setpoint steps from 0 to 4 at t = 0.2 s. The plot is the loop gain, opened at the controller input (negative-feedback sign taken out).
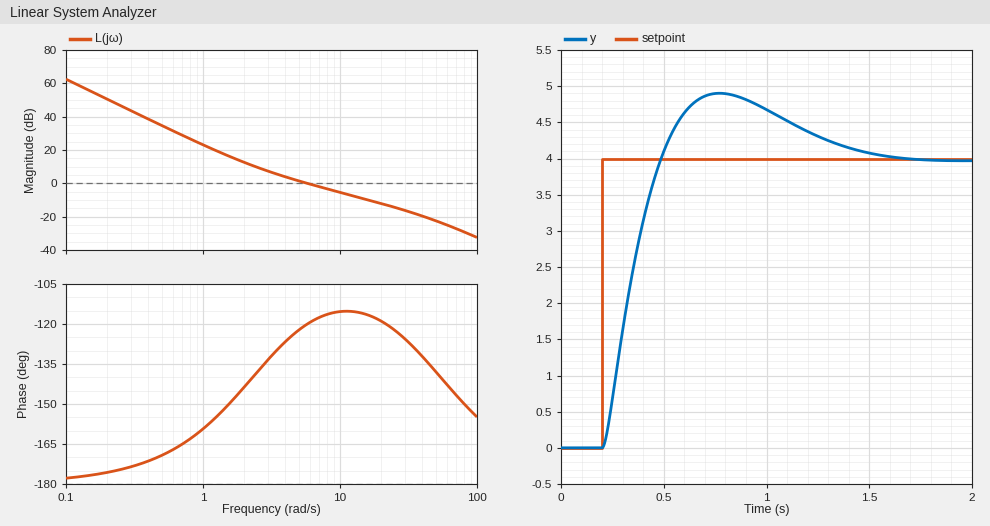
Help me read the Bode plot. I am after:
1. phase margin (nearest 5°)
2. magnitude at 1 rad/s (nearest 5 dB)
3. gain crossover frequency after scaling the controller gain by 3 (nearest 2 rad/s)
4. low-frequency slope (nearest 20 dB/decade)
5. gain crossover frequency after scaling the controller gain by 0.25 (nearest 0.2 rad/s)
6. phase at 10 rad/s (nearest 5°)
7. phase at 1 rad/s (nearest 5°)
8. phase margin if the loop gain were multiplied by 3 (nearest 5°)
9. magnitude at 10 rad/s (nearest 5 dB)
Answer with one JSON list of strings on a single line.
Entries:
["60°", "25 dB", "16 rad/s", "-40 dB/decade", "2.0 rad/s", "-115°", "-160°", "65°", "-5 dB"]
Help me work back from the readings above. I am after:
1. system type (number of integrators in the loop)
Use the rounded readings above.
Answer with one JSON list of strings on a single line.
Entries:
["2"]
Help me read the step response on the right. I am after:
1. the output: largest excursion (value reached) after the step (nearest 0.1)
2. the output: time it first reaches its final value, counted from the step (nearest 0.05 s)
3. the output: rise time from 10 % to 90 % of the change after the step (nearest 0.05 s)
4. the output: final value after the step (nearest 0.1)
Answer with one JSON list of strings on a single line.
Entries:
["4.9", "0.30 s", "0.20 s", "4.0"]
